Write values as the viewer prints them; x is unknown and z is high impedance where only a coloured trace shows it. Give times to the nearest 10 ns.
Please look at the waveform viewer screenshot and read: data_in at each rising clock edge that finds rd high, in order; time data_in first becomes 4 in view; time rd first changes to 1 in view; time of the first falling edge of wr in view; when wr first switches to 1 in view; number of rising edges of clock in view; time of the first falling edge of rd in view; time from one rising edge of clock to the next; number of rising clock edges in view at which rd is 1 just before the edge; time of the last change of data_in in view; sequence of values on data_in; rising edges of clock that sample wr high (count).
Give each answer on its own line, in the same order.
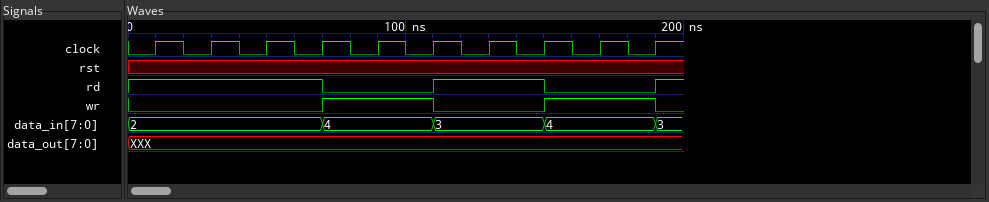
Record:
2, 2, 2, 2, 3, 3
70 ns
110 ns
110 ns
70 ns
10
70 ns
20 ns
6
190 ns
2, 4, 3, 4, 3
4
